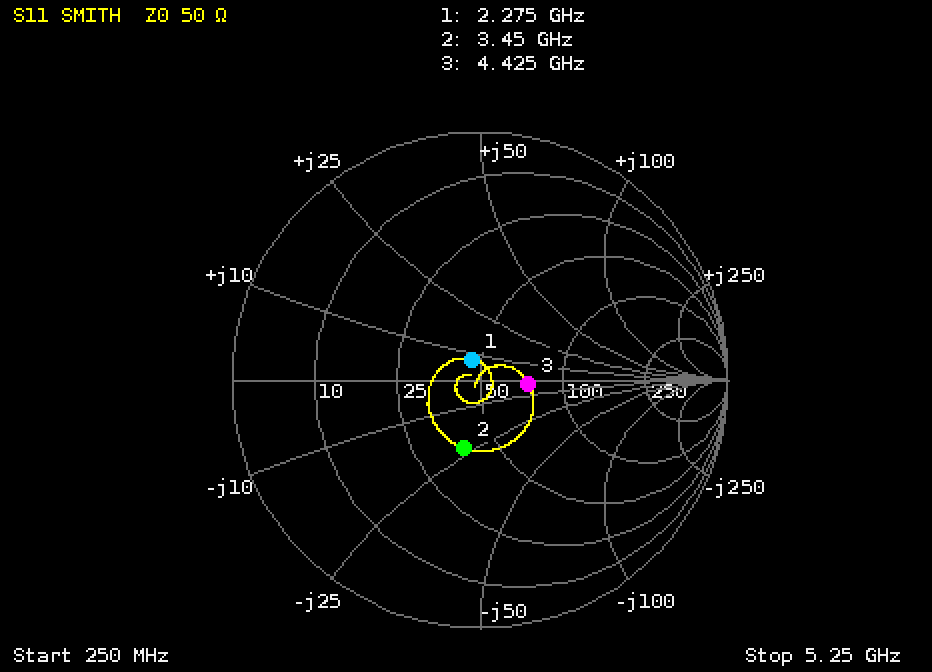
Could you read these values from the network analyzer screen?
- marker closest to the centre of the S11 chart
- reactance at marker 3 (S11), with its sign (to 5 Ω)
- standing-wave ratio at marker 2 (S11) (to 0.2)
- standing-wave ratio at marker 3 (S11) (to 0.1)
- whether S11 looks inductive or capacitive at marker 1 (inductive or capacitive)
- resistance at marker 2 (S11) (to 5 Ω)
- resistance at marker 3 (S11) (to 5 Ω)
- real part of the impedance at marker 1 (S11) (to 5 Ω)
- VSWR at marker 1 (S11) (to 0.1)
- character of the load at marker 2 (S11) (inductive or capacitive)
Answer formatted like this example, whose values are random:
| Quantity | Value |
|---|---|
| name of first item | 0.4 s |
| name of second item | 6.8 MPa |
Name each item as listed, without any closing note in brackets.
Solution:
| Quantity | Value |
|---|---|
| marker closest to the centre of the S11 chart | marker 1 |
| reactance at marker 3 (S11), with its sign | 0 Ω |
| standing-wave ratio at marker 2 (S11) | 1.8 |
| standing-wave ratio at marker 3 (S11) | 1.5 |
| whether S11 looks inductive or capacitive at marker 1 | inductive |
| resistance at marker 2 (S11) | 40 Ω |
| resistance at marker 3 (S11) | 75 Ω |
| real part of the impedance at marker 1 (S11) | 45 Ω |
| VSWR at marker 1 (S11) | 1.2 |
| character of the load at marker 2 (S11) | capacitive |
